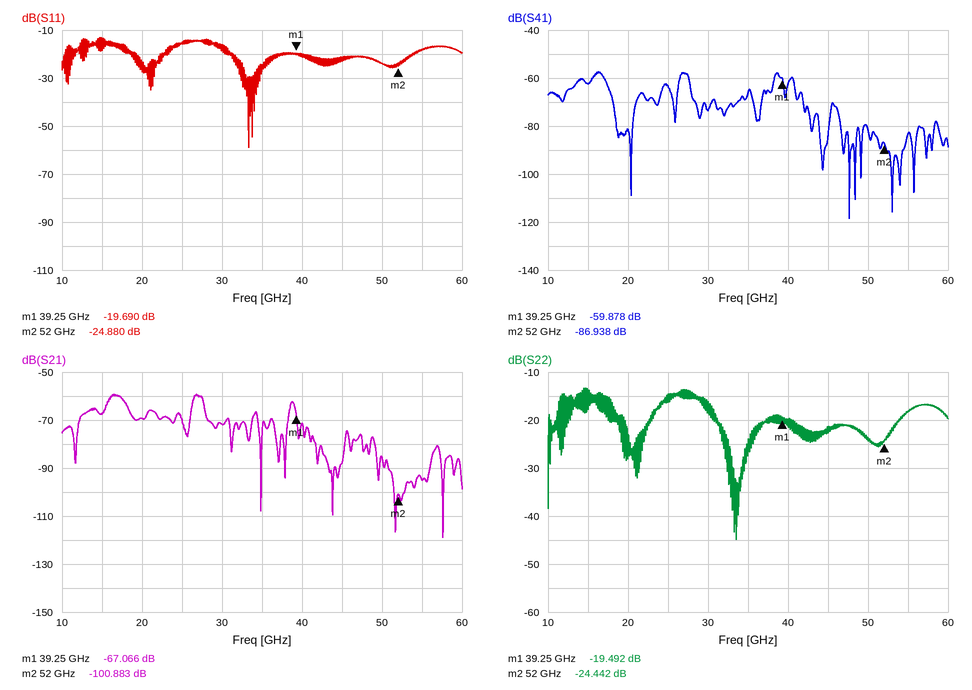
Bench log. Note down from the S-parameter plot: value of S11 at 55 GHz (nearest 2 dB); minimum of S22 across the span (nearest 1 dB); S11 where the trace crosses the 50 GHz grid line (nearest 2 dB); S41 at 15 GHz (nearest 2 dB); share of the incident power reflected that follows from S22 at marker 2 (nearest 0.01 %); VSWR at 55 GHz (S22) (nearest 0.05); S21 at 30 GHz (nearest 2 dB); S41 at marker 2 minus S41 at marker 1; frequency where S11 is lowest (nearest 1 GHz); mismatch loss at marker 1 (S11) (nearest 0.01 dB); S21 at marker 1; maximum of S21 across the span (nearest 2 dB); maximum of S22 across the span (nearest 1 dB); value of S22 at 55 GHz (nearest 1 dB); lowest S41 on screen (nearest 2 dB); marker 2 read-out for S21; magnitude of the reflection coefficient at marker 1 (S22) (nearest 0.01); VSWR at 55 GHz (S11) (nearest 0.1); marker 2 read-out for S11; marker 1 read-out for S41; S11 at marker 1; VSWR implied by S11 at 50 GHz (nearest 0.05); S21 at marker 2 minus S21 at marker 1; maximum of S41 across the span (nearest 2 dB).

-18 dB
-45 dB
-24 dB
-62 dB
0.36 %
1.30
-72 dB
-27.060 dB
33 GHz
0.05 dB
-67.066 dB
-60 dB
-13 dB
-18 dB
-118 dB
-100.883 dB
0.11
1.3
-24.880 dB
-59.878 dB
-19.690 dB
1.15
-33.817 dB
-58 dB
